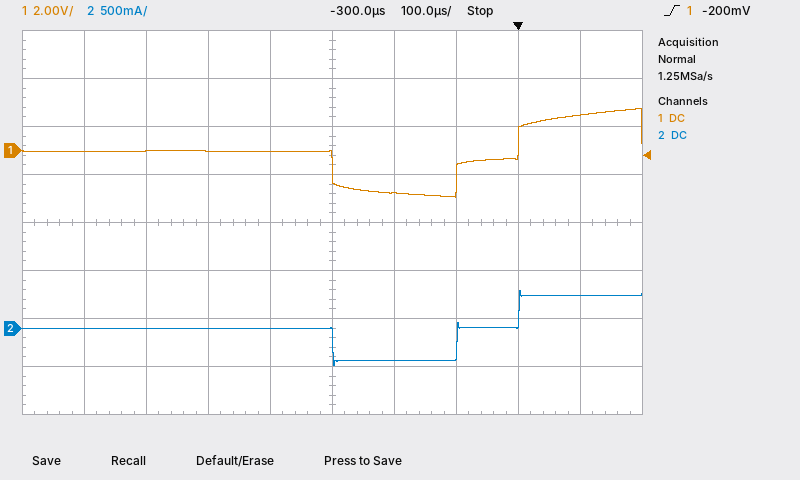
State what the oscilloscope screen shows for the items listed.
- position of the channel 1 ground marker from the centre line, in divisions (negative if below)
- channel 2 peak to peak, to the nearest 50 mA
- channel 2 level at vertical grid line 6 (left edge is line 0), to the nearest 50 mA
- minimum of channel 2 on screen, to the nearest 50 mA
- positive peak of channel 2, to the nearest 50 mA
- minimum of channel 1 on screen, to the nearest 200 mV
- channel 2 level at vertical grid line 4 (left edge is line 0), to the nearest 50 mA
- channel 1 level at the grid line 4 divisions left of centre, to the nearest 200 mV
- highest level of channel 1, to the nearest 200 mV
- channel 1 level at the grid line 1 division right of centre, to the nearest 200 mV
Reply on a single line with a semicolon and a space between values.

+1.5 div; 800 mA; -350 mA; -400 mA; 400 mA; -2.0 V; 0 mA; 0.0 V; 1.8 V; -1.8 V
